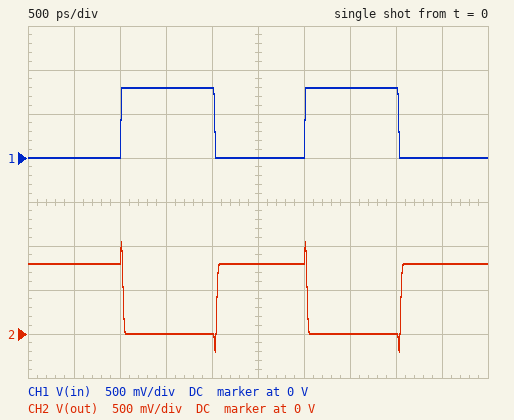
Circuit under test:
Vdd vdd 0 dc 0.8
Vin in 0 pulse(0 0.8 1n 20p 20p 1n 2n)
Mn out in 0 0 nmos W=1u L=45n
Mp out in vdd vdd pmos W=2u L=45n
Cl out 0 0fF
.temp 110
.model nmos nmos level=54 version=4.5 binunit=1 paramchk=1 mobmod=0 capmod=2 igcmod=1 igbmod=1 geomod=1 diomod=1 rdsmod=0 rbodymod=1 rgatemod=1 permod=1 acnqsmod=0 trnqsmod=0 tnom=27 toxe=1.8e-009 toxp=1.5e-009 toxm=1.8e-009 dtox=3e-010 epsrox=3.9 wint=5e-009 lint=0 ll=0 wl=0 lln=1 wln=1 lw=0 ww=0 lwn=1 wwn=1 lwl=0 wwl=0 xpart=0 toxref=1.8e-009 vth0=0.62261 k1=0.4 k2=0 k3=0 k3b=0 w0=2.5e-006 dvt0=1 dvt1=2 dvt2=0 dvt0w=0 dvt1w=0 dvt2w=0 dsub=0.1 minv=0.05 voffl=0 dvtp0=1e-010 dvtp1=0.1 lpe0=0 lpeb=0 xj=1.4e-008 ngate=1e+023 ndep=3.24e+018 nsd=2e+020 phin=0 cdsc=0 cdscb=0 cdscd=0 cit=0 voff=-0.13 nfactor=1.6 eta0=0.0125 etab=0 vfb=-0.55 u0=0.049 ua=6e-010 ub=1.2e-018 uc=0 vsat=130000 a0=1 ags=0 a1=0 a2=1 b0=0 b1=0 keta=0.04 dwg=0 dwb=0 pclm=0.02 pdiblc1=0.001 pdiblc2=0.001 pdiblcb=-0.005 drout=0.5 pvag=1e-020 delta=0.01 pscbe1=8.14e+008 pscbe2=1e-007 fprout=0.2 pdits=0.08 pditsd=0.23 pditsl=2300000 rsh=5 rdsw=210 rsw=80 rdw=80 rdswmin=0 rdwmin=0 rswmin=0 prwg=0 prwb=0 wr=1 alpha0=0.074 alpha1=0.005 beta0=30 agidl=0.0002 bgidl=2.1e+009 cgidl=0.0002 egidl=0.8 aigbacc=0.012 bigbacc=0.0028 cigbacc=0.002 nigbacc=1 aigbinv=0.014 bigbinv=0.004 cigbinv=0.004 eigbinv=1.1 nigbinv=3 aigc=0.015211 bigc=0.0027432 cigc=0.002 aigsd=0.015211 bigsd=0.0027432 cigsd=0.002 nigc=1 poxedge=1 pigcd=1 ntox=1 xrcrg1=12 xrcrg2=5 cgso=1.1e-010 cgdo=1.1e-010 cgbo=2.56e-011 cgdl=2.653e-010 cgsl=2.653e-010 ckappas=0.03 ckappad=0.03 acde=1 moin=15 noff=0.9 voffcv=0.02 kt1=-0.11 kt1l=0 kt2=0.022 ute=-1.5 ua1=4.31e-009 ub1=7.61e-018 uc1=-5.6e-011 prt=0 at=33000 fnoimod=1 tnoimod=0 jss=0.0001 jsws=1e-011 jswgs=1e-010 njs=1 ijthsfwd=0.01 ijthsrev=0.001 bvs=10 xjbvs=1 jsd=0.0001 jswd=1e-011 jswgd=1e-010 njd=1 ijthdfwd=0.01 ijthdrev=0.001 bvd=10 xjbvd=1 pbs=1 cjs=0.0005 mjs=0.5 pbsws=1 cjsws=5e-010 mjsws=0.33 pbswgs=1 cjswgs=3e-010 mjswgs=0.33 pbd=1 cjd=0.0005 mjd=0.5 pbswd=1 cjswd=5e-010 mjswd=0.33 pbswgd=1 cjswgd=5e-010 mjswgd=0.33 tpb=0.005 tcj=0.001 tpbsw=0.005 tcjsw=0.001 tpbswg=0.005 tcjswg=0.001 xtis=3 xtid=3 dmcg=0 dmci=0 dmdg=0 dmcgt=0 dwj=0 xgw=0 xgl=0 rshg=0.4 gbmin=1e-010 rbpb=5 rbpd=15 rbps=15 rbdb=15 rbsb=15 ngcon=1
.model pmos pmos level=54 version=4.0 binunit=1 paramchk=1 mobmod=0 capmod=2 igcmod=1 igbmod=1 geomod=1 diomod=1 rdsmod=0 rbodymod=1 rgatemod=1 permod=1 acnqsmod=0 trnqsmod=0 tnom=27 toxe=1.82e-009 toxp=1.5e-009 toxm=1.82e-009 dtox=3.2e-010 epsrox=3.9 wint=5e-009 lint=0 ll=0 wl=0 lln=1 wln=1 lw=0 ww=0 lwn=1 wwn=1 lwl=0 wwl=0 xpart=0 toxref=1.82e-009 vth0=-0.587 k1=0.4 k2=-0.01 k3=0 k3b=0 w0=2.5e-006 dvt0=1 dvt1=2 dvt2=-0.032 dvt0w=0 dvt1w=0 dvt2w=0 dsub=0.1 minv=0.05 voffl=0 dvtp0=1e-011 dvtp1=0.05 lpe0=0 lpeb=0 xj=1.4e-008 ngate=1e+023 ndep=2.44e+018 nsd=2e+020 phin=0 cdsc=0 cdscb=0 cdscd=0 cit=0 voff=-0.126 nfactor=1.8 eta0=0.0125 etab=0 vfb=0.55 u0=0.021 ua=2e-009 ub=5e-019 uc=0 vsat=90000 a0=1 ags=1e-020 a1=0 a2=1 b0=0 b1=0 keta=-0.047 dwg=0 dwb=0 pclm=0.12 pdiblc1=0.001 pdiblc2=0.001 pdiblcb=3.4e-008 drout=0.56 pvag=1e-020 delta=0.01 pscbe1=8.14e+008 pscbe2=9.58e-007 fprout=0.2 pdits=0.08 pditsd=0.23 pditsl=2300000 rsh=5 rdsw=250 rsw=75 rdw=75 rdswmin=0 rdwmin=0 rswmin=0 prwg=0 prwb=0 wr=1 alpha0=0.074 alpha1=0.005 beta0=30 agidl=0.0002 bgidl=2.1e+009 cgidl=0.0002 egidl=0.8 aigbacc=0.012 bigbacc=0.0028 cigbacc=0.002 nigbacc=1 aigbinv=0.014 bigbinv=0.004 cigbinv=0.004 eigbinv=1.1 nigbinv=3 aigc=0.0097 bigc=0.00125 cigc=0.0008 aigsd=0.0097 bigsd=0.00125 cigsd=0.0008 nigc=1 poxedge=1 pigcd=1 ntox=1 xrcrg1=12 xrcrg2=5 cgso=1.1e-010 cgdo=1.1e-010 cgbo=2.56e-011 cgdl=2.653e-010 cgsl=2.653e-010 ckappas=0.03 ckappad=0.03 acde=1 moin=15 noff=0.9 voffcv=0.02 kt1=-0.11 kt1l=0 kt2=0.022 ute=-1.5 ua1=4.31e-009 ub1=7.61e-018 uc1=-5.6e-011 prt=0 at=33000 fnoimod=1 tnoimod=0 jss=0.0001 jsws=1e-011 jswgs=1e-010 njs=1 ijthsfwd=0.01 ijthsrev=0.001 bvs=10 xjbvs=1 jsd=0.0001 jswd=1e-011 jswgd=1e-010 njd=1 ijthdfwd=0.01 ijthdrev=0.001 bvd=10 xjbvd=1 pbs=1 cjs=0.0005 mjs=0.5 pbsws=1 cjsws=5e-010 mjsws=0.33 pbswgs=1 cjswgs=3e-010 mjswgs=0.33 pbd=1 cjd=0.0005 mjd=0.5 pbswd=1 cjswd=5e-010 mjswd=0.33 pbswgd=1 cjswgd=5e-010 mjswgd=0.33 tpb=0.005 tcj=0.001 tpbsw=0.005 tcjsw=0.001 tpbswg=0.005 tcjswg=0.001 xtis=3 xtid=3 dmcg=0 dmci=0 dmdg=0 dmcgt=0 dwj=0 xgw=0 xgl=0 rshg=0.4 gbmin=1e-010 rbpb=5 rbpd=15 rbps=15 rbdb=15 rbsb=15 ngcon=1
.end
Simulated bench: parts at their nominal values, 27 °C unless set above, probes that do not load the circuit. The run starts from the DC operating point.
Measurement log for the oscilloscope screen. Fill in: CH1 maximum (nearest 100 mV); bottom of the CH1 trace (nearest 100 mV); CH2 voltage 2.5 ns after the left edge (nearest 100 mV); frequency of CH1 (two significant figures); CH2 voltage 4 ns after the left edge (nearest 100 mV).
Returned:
800 mV
0 V
800 mV
500 MHz
0 V
